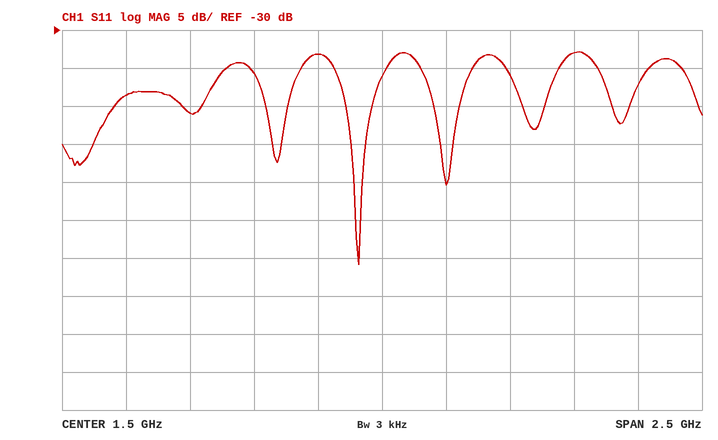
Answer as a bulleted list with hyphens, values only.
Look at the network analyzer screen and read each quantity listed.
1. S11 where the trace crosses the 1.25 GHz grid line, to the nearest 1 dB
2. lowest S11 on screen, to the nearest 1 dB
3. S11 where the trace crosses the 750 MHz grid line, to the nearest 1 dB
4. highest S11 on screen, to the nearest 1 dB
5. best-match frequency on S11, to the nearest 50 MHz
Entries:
- -33 dB
- -61 dB
- -41 dB
- -33 dB
- 1.40 GHz
